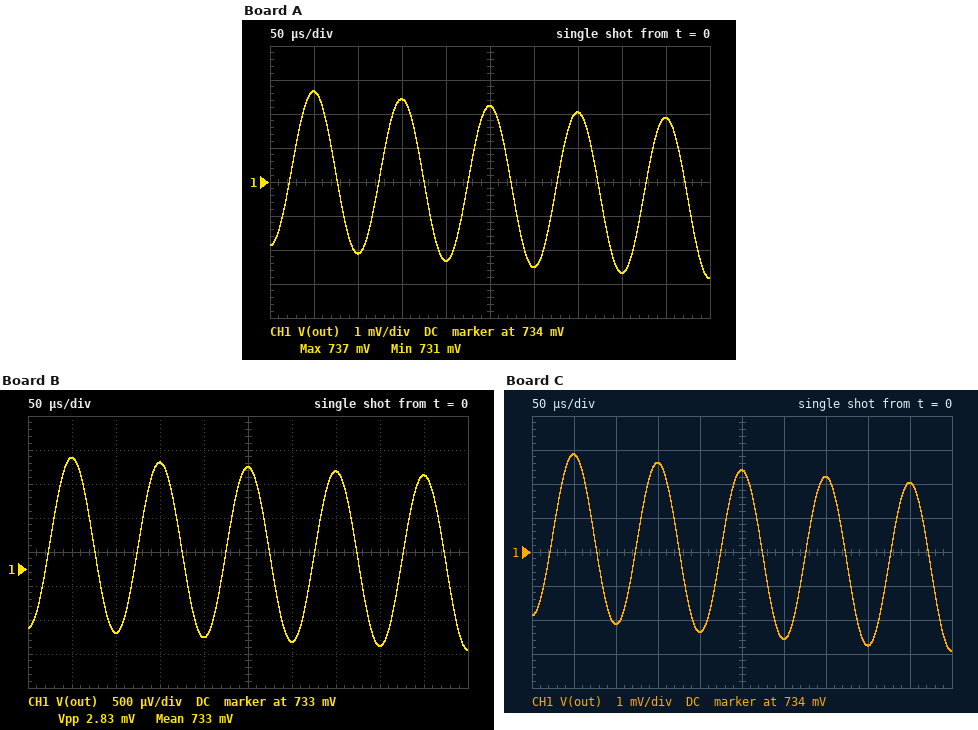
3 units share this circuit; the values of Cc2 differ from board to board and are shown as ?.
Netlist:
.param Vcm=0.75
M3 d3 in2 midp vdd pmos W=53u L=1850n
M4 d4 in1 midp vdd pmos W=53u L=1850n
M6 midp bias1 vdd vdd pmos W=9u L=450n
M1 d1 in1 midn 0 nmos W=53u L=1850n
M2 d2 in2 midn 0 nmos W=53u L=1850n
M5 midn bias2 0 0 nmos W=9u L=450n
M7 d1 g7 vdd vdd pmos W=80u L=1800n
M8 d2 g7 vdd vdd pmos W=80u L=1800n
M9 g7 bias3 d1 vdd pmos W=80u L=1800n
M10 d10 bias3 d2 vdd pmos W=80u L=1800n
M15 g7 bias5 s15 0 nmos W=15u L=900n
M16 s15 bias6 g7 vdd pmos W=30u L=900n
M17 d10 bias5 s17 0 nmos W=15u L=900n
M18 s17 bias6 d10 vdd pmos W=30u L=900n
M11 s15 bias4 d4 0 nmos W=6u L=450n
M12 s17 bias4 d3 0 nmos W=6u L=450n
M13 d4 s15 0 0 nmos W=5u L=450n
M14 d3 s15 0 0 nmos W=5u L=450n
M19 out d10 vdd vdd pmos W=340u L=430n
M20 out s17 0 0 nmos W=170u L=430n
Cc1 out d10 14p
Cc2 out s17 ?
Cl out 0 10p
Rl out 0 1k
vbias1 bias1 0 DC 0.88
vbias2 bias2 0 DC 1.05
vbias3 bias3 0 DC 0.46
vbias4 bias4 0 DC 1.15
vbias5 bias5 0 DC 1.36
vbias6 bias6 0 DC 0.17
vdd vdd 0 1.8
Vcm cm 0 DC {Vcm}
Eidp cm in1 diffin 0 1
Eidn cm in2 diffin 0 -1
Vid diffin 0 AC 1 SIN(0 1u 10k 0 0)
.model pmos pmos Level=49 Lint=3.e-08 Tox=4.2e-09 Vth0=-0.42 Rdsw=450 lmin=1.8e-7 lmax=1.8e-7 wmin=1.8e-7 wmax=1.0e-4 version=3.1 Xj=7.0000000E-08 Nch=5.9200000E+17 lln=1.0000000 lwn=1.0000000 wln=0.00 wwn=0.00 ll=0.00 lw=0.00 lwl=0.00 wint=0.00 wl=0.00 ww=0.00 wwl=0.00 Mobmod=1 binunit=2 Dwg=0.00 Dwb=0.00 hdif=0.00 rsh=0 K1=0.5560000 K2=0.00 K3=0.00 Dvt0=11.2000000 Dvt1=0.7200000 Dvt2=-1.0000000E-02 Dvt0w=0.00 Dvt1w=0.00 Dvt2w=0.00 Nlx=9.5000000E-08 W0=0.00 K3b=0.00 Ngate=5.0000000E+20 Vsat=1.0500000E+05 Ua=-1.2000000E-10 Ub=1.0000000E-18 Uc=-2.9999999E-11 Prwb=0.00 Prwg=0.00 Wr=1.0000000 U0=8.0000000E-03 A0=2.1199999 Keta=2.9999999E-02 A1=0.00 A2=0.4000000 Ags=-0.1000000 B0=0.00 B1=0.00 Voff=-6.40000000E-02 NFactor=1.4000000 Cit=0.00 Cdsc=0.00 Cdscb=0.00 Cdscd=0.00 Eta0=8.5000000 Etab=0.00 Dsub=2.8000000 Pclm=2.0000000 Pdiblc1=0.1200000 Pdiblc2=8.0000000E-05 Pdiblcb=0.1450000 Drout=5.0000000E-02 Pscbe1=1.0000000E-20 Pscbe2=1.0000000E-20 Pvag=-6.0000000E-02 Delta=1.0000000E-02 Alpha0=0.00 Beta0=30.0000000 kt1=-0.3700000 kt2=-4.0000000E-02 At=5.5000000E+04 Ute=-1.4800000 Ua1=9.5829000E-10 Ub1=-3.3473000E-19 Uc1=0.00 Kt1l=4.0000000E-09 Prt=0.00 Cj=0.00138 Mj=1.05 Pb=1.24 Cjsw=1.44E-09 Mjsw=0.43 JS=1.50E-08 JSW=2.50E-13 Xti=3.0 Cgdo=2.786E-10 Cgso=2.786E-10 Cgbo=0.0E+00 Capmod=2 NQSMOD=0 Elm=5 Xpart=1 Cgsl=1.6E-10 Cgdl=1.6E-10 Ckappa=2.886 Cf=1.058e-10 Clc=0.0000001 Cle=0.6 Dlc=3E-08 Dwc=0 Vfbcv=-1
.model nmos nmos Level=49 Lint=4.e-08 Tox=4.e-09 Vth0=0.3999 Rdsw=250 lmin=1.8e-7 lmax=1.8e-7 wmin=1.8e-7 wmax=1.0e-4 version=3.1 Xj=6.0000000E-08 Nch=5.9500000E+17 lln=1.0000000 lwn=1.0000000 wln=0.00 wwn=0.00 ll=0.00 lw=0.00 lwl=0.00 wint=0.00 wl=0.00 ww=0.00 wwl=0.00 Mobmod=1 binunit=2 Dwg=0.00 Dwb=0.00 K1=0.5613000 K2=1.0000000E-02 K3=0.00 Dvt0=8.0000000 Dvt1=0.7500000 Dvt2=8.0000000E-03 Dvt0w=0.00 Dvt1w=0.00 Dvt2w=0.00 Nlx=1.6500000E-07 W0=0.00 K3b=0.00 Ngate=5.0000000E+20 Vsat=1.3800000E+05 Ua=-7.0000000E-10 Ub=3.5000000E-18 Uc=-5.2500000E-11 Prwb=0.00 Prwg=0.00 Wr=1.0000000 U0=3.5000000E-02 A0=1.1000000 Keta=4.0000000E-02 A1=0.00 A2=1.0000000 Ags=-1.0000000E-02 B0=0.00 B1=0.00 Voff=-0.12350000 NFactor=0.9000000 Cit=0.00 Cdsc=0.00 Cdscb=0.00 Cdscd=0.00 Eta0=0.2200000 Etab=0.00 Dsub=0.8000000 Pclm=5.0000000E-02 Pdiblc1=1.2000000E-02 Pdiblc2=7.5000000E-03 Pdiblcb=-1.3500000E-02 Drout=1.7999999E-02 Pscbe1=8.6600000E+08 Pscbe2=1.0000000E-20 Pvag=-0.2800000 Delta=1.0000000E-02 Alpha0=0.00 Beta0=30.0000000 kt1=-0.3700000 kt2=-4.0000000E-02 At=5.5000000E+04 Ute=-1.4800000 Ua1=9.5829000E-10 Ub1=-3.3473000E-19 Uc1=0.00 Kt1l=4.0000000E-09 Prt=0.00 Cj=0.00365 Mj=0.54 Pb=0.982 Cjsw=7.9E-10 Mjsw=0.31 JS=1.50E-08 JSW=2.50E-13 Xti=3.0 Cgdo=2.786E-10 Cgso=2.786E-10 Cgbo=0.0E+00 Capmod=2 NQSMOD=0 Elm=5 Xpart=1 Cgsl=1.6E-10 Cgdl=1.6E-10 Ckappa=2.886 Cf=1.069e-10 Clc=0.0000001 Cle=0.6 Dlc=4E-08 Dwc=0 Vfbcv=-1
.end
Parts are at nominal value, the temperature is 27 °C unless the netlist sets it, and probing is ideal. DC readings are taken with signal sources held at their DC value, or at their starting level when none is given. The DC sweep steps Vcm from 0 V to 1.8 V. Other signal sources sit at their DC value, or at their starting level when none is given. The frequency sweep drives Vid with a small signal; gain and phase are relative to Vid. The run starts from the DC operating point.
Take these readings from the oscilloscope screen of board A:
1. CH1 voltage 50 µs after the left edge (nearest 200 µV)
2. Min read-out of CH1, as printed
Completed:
736.6 mV
731 mV
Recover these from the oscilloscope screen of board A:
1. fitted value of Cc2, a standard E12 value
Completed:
5.6 pF
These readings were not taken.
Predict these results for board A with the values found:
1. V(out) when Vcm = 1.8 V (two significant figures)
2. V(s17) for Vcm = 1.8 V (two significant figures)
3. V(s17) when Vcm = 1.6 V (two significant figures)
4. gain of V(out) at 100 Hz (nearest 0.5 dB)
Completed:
1.7 V
630 mV
630 mV
101.5 dB
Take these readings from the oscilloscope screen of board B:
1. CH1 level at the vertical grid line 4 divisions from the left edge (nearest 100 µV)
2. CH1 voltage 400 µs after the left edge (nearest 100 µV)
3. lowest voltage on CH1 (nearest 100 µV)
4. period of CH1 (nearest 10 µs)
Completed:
732.0 mV
731.9 mV
731.8 mV
100 µs
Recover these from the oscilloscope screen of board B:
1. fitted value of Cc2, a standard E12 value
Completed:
22 pF
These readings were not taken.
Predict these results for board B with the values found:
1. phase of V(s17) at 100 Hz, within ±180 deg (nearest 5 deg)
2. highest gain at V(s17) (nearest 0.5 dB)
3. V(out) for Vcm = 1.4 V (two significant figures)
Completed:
135 deg
79.5 dB
1.7 V
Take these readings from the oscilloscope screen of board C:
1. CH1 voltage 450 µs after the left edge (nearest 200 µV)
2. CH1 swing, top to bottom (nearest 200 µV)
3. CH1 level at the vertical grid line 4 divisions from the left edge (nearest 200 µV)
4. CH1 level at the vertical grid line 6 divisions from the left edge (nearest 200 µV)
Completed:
736.0 mV
5.8 mV
731.6 mV
731.4 mV
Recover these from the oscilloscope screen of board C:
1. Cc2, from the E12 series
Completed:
4.7 pF
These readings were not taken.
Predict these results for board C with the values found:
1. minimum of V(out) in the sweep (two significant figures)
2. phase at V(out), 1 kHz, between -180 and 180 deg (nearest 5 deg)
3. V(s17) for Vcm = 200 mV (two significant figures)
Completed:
52 mV
-80 deg
800 mV
